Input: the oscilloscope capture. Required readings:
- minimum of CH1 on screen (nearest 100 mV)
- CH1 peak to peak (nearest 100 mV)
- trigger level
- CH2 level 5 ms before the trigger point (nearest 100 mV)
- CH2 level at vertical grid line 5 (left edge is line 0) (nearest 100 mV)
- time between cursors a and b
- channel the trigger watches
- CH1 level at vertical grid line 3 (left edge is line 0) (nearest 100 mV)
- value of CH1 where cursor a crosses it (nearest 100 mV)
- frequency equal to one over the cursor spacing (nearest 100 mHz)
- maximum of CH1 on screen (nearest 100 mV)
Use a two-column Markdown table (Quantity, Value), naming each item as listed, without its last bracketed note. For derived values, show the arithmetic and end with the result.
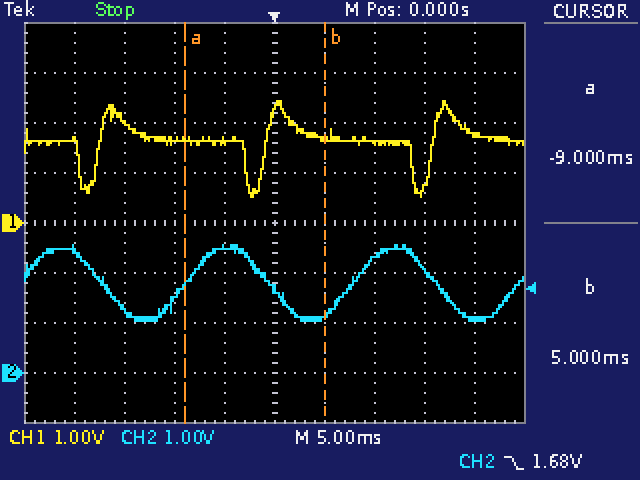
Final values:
| Quantity | Value |
|---|---|
| minimum of CH1 on screen | 500 mV |
| CH1 peak to peak | 2.4 V − (500 mV) = 1.9 V |
| trigger level | 1.68 V |
| CH2 level 5 ms before the trigger point | 2.5 V |
| CH2 level at vertical grid line 5 (left edge is line 0) | 1.7 V |
| time between cursors a and b | 5 ms − (-9 ms) = 14.0 ms |
| channel the trigger watches | CH2 |
| CH1 level at vertical grid line 3 (left edge is line 0) | 1.6 V |
| value of CH1 where cursor a crosses it | 1.6 V |
| frequency equal to one over the cursor spacing | 1 / 14.0 ms ≈ 71.4 Hz |
| maximum of CH1 on screen | 2.4 V |
